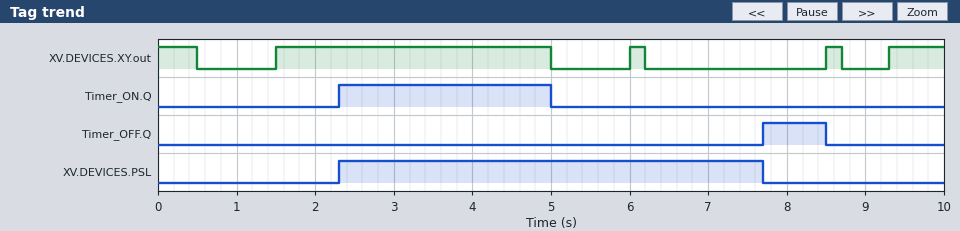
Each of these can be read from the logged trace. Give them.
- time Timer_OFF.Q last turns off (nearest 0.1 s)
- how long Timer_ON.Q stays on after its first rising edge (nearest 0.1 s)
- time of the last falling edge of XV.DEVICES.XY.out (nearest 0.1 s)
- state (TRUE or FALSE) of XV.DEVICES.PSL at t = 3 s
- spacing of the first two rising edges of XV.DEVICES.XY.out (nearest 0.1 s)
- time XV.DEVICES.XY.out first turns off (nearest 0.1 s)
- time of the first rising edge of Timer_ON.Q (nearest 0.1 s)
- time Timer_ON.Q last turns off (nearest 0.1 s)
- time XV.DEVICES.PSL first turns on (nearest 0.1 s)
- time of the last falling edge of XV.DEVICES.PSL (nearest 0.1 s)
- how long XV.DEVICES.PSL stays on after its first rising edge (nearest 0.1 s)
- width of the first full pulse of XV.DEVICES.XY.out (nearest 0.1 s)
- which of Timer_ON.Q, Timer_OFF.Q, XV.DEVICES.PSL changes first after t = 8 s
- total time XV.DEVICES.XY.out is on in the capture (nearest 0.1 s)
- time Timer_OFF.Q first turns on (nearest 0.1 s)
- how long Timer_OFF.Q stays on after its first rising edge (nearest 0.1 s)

8.5 s
2.7 s
8.7 s
TRUE
4.5 s
0.5 s
2.3 s
5.0 s
2.3 s
7.7 s
5.4 s
3.5 s
Timer_OFF.Q
5.1 s
7.7 s
0.8 s
